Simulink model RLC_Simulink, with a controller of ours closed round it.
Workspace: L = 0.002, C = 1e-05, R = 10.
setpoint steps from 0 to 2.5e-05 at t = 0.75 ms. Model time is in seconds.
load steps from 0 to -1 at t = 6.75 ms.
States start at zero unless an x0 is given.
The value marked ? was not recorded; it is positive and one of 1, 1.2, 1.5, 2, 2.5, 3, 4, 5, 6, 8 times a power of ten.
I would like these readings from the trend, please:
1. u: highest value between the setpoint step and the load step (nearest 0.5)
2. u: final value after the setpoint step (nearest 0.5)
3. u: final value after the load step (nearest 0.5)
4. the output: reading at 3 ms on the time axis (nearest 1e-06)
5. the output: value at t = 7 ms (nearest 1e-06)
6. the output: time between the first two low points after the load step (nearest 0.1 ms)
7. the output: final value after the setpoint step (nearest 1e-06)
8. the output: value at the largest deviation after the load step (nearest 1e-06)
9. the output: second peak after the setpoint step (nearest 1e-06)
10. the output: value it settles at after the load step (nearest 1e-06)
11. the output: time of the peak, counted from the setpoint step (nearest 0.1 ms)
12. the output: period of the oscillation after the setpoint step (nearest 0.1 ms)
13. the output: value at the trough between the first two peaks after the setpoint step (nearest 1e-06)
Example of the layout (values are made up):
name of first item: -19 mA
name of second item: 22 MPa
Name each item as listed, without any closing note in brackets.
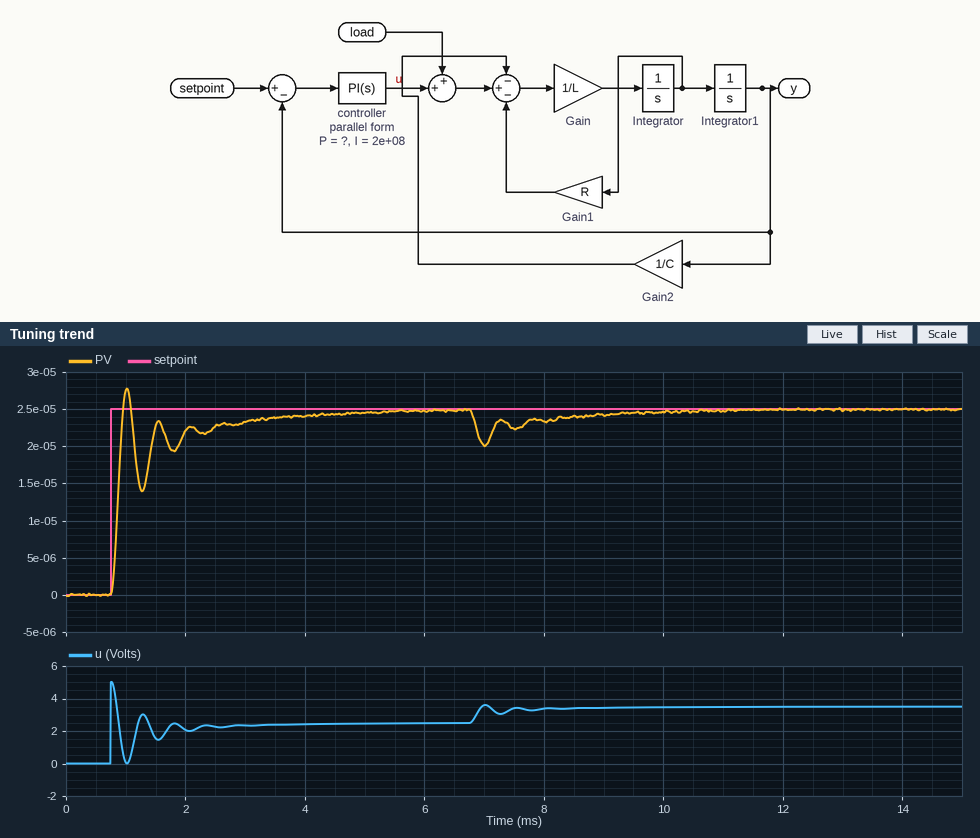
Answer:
u: highest value between the setpoint step and the load step: 5.0
u: final value after the setpoint step: 2.5
u: final value after the load step: 3.5
the output: reading at 3 ms on the time axis: 0.000023
the output: value at t = 7 ms: 0.000020
the output: time between the first two low points after the load step: 0.5 ms
the output: final value after the setpoint step: 0.000025
the output: value at the largest deviation after the load step: 0.000020
the output: second peak after the setpoint step: 0.000023
the output: value it settles at after the load step: 0.000025
the output: time of the peak, counted from the setpoint step: 0.3 ms
the output: period of the oscillation after the setpoint step: 0.5 ms
the output: value at the trough between the first two peaks after the setpoint step: 0.000014
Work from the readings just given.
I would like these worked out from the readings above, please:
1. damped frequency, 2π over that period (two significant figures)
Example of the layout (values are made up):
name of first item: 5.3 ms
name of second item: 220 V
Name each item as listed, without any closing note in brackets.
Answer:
damped frequency, 2π over that period: 13 rad/ms
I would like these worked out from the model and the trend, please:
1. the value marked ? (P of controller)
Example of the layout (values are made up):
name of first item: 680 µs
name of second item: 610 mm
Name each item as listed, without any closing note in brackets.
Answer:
the value marked ?: 200000
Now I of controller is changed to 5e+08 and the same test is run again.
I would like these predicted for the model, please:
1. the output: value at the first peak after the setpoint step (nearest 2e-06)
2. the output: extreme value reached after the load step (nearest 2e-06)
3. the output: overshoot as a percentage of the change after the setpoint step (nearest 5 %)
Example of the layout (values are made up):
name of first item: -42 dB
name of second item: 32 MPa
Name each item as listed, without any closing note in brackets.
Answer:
the output: value at the first peak after the setpoint step: 0.000032
the output: extreme value reached after the load step: 0.000020
the output: overshoot as a percentage of the change after the setpoint step: 25 %
